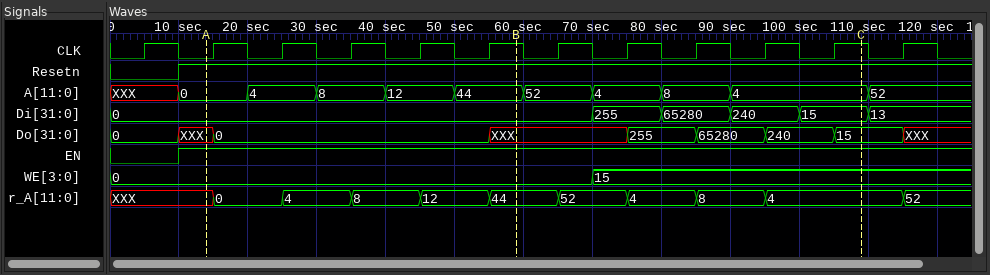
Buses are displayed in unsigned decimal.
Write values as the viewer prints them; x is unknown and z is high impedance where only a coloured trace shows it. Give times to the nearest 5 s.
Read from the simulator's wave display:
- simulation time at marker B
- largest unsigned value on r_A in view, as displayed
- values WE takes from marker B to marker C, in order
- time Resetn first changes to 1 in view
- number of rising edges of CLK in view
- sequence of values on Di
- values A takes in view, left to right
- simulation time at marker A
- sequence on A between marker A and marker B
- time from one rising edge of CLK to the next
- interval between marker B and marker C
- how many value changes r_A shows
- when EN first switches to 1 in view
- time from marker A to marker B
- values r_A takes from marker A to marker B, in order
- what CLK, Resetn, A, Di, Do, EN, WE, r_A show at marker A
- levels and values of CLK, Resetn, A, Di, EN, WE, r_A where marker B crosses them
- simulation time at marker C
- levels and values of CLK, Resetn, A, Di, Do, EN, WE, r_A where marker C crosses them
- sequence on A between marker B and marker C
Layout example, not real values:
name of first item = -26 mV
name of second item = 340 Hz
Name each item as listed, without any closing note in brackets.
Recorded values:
simulation time at marker B = 60 s
largest unsigned value on r_A in view, as displayed = 52
values WE takes from marker B to marker C, in order = 0, 15
time Resetn first changes to 1 in view = 10 s
number of rising edges of CLK in view = 12
sequence of values on Di = 0, 255, 65280, 240, 15, 13
values A takes in view, left to right = XXX, 0, 4, 8, 12, 44, 52, 4, 8, 4, 52
simulation time at marker A = 15 s
sequence on A between marker A and marker B = 0, 4, 8, 12, 44
time from one rising edge of CLK to the next = 10 s
interval between marker B and marker C = 50 s
how many value changes r_A shows = 10
when EN first switches to 1 in view = 10 s
time from marker A to marker B = 45 s
values r_A takes from marker A to marker B, in order = XXX, 0, 4, 8, 12, 44
what CLK, Resetn, A, Di, Do, EN, WE, r_A show at marker A = CLK=0, Resetn=1, A=0, Di=0, Do=XXX, EN=1, WE=0, r_A=XXX
levels and values of CLK, Resetn, A, Di, EN, WE, r_A where marker B crosses them = CLK=1, Resetn=1, A=44, Di=0, EN=1, WE=0, r_A=44
simulation time at marker C = 110 s
levels and values of CLK, Resetn, A, Di, Do, EN, WE, r_A where marker C crosses them = CLK=1, Resetn=1, A=4, Di=15, Do=15, EN=1, WE=15, r_A=4
sequence on A between marker B and marker C = 44, 52, 4, 8, 4
